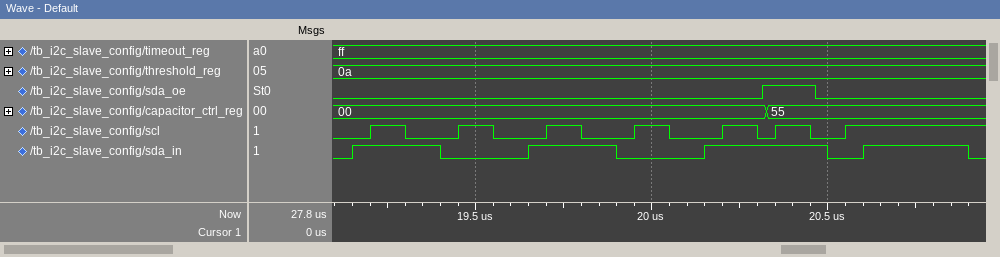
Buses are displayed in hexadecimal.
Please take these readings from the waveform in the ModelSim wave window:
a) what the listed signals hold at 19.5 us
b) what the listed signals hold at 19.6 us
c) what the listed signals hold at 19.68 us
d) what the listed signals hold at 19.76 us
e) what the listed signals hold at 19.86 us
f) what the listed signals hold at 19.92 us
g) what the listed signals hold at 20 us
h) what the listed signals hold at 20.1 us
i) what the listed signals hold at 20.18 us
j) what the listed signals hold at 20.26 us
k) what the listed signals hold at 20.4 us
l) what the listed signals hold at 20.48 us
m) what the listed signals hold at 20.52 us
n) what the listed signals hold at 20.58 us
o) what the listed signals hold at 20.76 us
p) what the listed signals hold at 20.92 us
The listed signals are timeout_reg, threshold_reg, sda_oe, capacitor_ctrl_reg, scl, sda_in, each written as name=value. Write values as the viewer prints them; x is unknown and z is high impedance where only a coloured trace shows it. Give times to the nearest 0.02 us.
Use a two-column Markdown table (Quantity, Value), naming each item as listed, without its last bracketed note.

| Quantity | Value |
|---|---|
| what the listed signals hold at 19.5 us | timeout_reg=ff, threshold_reg=0a, sda_oe=0, capacitor_ctrl_reg=00, scl=1, sda_in=0 |
| what the listed signals hold at 19.6 us | timeout_reg=ff, threshold_reg=0a, sda_oe=0, capacitor_ctrl_reg=00, scl=0, sda_in=0 |
| what the listed signals hold at 19.68 us | timeout_reg=ff, threshold_reg=0a, sda_oe=0, capacitor_ctrl_reg=00, scl=0, sda_in=1 |
| what the listed signals hold at 19.76 us | timeout_reg=ff, threshold_reg=0a, sda_oe=0, capacitor_ctrl_reg=00, scl=1, sda_in=1 |
| what the listed signals hold at 19.86 us | timeout_reg=ff, threshold_reg=0a, sda_oe=0, capacitor_ctrl_reg=00, scl=0, sda_in=1 |
| what the listed signals hold at 19.92 us | timeout_reg=ff, threshold_reg=0a, sda_oe=0, capacitor_ctrl_reg=00, scl=0, sda_in=0 |
| what the listed signals hold at 20 us | timeout_reg=ff, threshold_reg=0a, sda_oe=0, capacitor_ctrl_reg=00, scl=1, sda_in=0 |
| what the listed signals hold at 20.1 us | timeout_reg=ff, threshold_reg=0a, sda_oe=0, capacitor_ctrl_reg=00, scl=0, sda_in=0 |
| what the listed signals hold at 20.18 us | timeout_reg=ff, threshold_reg=0a, sda_oe=0, capacitor_ctrl_reg=00, scl=0, sda_in=1 |
| what the listed signals hold at 20.26 us | timeout_reg=ff, threshold_reg=0a, sda_oe=0, capacitor_ctrl_reg=00, scl=1, sda_in=1 |
| what the listed signals hold at 20.4 us | timeout_reg=ff, threshold_reg=0a, sda_oe=1, capacitor_ctrl_reg=55, scl=1, sda_in=1 |
| what the listed signals hold at 20.48 us | timeout_reg=ff, threshold_reg=0a, sda_oe=0, capacitor_ctrl_reg=55, scl=0, sda_in=1 |
| what the listed signals hold at 20.52 us | timeout_reg=ff, threshold_reg=0a, sda_oe=0, capacitor_ctrl_reg=55, scl=0, sda_in=0 |
| what the listed signals hold at 20.58 us | timeout_reg=ff, threshold_reg=0a, sda_oe=0, capacitor_ctrl_reg=55, scl=1, sda_in=0 |
| what the listed signals hold at 20.76 us | timeout_reg=ff, threshold_reg=0a, sda_oe=0, capacitor_ctrl_reg=55, scl=1, sda_in=1 |
| what the listed signals hold at 20.92 us | timeout_reg=ff, threshold_reg=0a, sda_oe=0, capacitor_ctrl_reg=55, scl=1, sda_in=0 |
